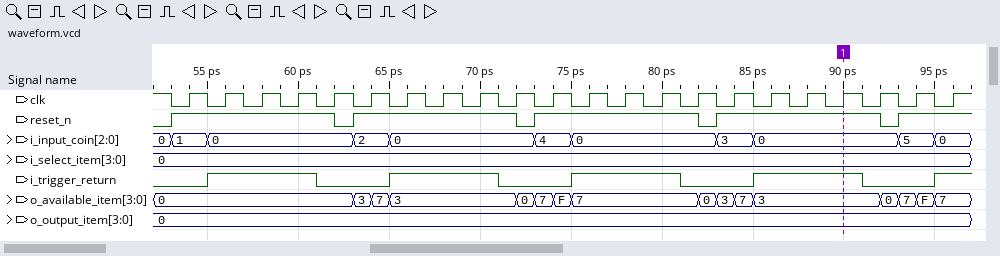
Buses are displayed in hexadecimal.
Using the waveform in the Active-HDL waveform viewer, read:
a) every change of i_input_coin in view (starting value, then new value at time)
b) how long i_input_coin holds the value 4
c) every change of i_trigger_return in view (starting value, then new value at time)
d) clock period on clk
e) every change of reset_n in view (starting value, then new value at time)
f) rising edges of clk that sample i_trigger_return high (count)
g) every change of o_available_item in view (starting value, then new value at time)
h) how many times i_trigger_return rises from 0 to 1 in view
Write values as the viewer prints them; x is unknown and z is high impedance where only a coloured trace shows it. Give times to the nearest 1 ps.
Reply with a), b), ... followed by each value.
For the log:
a) 0, 1 at 53 ps, 0 at 55 ps, 2 at 63 ps, 0 at 65 ps, 4 at 73 ps, 0 at 75 ps, 3 at 83 ps, 0 at 85 ps, 5 at 93 ps, 0 at 95 ps
b) 2 ps
c) 0, 1 at 55 ps, 0 at 61 ps, 1 at 65 ps, 0 at 71 ps, 1 at 75 ps, 0 at 81 ps, 1 at 85 ps, 0 at 91 ps, 1 at 95 ps
d) 2 ps
e) 0, 1 at 53 ps, 0 at 62 ps, 1 at 63 ps, 0 at 72 ps, 1 at 73 ps, 0 at 82 ps, 1 at 83 ps, 0 at 92 ps, 1 at 93 ps
f) 13
g) 0, 3 at 63 ps, 7 at 64 ps, 3 at 65 ps, 0 at 72 ps, 7 at 73 ps, F at 74 ps, 7 at 75 ps, 0 at 82 ps, 3 at 83 ps, 7 at 84 ps, 3 at 85 ps, 0 at 92 ps, 7 at 93 ps, F at 94 ps, 7 at 95 ps
h) 5
